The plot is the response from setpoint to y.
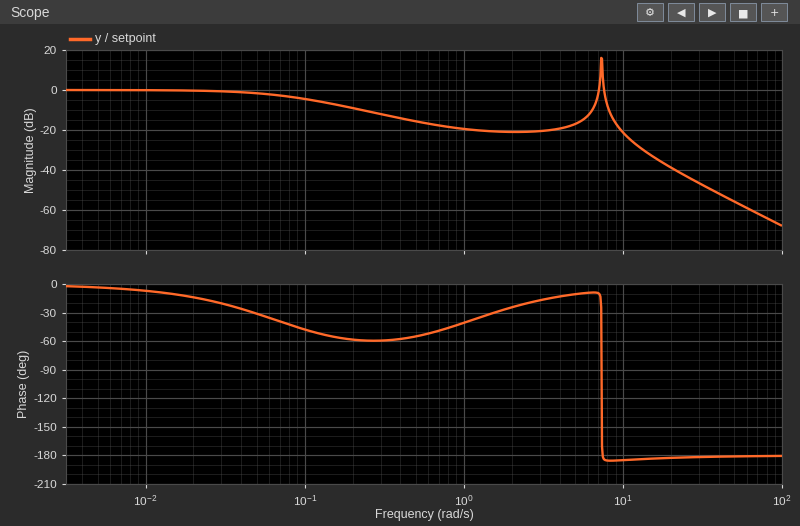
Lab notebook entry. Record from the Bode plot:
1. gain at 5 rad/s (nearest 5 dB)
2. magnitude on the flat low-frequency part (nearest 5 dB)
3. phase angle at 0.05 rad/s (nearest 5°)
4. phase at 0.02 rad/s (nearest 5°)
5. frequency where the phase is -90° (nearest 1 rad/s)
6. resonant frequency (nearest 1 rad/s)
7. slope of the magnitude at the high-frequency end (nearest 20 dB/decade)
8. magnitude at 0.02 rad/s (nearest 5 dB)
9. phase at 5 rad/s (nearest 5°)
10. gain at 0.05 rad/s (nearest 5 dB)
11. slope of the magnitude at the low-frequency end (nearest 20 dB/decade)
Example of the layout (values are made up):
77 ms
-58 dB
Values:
-15 dB
0 dB
-30°
-15°
7 rad/s
7 rad/s
-40 dB/decade
0 dB
-10°
0 dB
0 dB/decade
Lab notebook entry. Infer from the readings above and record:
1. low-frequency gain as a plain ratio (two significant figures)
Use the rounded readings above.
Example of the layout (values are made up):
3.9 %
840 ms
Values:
1.0
